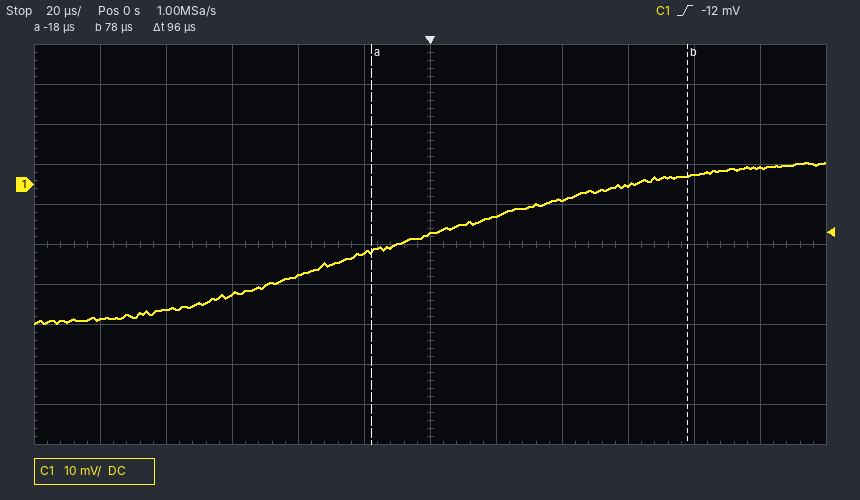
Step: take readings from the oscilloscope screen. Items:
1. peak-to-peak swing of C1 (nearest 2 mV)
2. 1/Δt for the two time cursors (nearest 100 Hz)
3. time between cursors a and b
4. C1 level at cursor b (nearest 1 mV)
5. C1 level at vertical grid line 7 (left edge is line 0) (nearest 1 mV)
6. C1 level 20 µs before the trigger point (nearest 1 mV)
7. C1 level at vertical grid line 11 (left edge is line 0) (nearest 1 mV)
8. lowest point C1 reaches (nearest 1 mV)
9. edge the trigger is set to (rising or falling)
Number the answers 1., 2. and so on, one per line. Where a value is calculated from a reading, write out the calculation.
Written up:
1. 40 mV
2. 1 / 96 µs ≈ 10.4 kHz
3. 96 µs
4. 2 mV
5. -8 mV
6. -17 mV
7. 4 mV
8. -35 mV
9. rising
